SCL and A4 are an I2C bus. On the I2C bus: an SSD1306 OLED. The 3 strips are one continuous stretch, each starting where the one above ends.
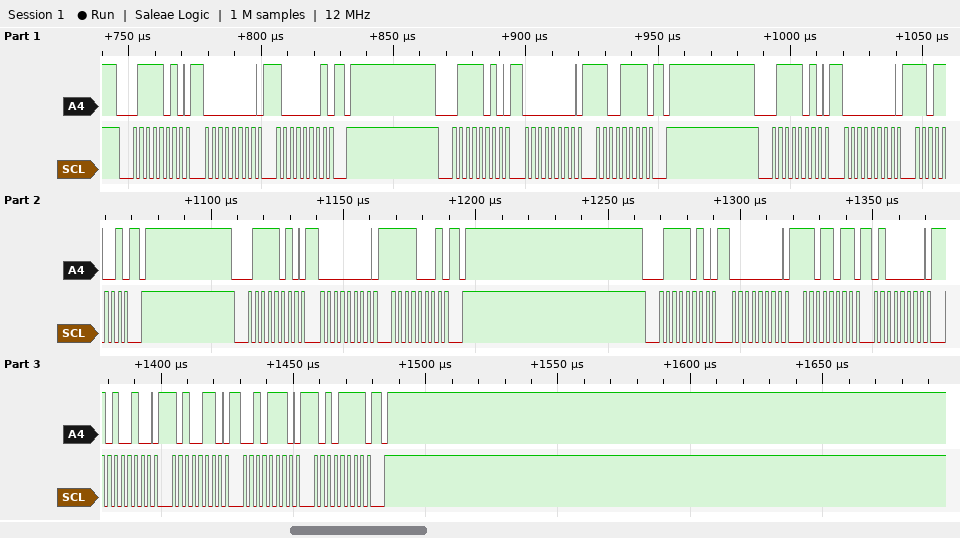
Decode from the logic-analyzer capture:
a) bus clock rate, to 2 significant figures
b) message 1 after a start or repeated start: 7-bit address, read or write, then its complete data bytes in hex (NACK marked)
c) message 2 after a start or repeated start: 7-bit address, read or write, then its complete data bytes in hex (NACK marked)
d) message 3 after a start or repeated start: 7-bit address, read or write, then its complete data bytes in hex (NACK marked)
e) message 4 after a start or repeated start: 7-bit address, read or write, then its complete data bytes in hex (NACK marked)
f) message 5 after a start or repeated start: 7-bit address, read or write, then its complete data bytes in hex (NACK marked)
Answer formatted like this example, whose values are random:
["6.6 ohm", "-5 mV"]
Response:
["400 kHz", "0x3D write: 00 81", "0x3D write: 00 CF", "0x3D write: 00 D9", "0x3D write: 00 F1", "0x3D write: 00 DB 40 A4 A6 2E AF"]
